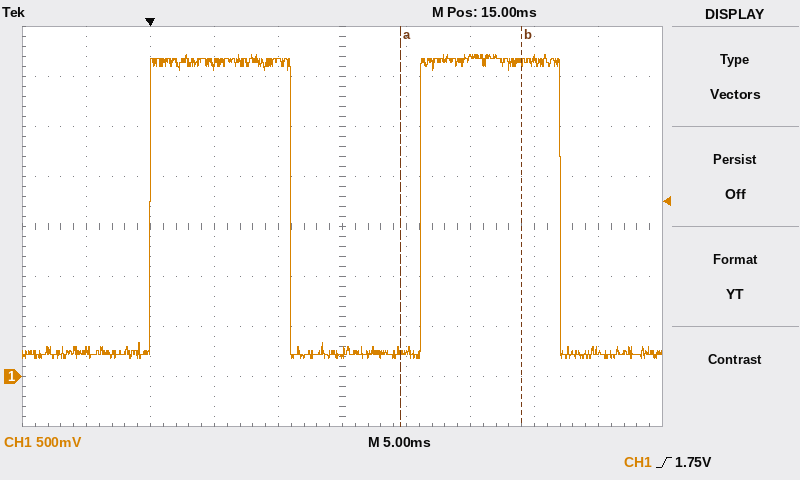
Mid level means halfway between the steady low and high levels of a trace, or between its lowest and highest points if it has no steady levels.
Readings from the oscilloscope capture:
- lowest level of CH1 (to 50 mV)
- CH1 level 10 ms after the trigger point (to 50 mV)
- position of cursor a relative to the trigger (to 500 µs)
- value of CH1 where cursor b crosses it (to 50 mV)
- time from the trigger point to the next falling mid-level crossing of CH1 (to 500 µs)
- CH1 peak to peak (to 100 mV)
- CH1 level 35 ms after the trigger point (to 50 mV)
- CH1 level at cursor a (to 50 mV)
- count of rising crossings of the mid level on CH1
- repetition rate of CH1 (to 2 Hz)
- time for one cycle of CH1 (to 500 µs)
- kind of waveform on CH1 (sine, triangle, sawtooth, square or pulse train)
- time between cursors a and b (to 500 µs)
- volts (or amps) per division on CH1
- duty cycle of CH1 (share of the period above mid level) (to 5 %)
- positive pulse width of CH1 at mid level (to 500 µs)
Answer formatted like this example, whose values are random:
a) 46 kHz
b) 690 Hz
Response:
a) 200 mV
b) 3.15 V
c) +19.5 ms
d) 3.15 V
e) 11.0 ms
f) 3.00 V
g) 250 mV
h) 250 mV
i) 2
j) 48 Hz
k) 21.0 ms
l) square
m) 9.5 ms
n) 500 mV
o) 50 %
p) 11.0 ms
